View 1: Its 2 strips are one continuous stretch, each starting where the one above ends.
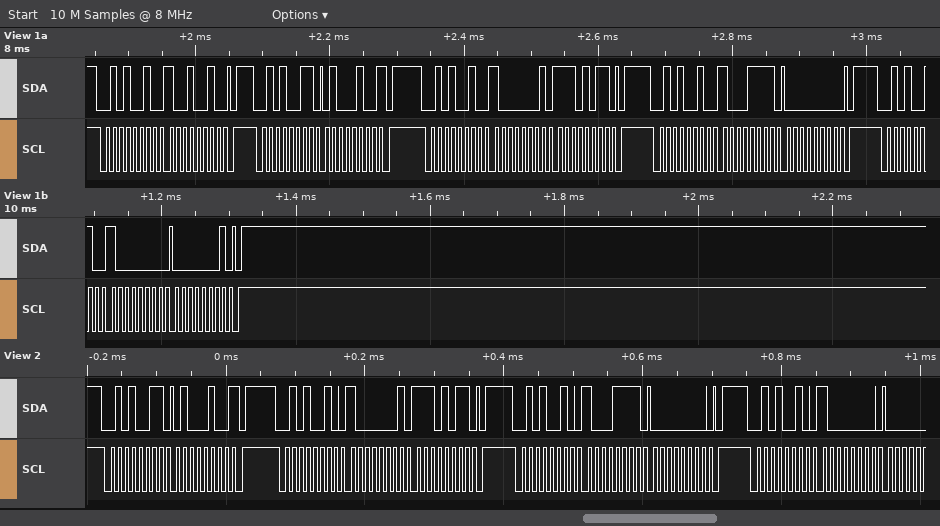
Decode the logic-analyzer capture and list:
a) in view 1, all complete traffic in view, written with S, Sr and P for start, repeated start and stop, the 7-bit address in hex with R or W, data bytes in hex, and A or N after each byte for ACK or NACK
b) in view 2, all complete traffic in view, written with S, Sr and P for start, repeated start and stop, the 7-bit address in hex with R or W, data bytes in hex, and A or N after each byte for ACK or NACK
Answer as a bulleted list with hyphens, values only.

- S 29W A 92 A P S 29R A 44 N P S 29W A 81 A EB A P S 29W A 8F A 00 A P S 29W A 80 A 01 A P
- S 29R A 44 N P S 29W A 81 A EB A P S 29W A 8F A 00 A P S 29W A 80 A
